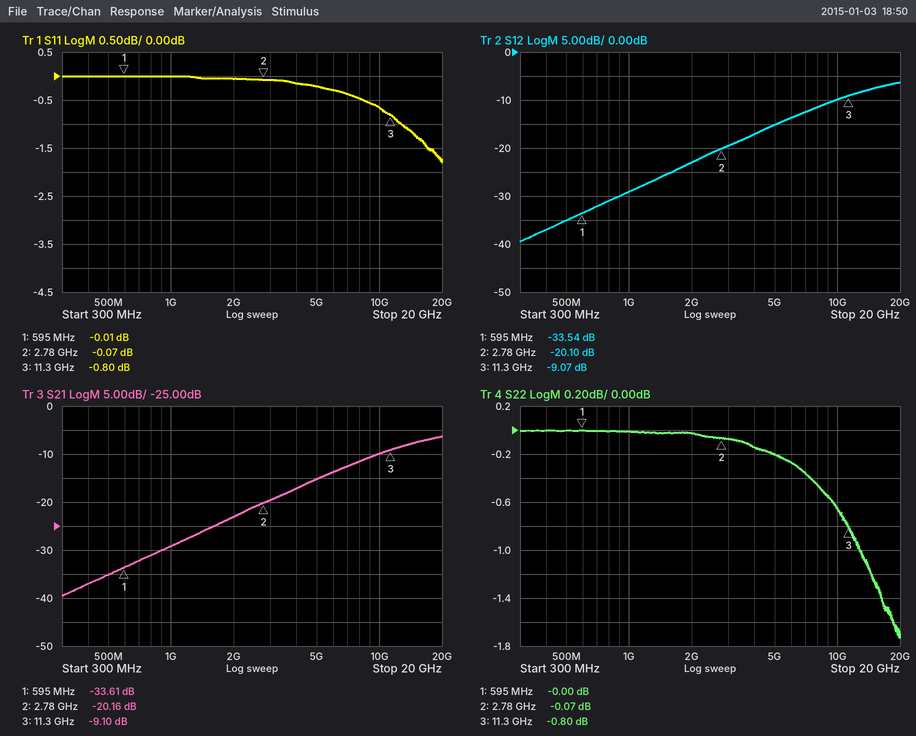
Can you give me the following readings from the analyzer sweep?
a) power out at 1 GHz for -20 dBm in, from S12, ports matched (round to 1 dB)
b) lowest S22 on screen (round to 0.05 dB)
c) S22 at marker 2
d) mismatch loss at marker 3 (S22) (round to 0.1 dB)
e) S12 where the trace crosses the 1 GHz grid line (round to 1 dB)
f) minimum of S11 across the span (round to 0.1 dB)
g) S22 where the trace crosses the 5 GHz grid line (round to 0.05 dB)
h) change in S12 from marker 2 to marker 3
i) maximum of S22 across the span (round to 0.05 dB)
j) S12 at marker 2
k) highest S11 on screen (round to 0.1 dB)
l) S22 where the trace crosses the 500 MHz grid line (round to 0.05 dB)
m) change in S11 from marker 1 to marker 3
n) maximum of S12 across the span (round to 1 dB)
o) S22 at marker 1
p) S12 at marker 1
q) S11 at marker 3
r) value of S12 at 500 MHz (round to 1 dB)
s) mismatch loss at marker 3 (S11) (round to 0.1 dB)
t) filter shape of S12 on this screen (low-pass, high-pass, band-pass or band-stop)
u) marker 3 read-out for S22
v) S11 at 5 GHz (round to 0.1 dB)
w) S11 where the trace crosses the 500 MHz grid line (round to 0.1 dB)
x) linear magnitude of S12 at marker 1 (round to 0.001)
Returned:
-49 dBm
-1.75 dB
-0.07 dB
7.7 dB
-29 dB
-1.8 dB
-0.20 dB
11.03 dB
0.00 dB
-20.10 dB
0.0 dB
0.00 dB
-0.79 dB
-6 dB
-0.00 dB
-33.54 dB
-0.80 dB
-35 dB
7.7 dB
high-pass
-0.80 dB
-0.2 dB
0.0 dB
0.021
